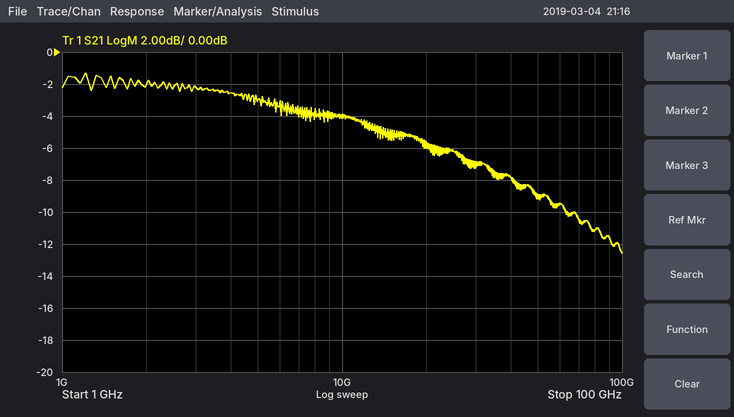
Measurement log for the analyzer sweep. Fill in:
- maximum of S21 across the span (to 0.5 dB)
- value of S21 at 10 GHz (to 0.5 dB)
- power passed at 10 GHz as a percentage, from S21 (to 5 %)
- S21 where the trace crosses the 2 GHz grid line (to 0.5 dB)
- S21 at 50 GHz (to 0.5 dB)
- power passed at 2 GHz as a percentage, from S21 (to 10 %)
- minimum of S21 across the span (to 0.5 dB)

-1.5 dB
-4.0 dB
40 %
-2.0 dB
-9.0 dB
60 %
-12.5 dB
